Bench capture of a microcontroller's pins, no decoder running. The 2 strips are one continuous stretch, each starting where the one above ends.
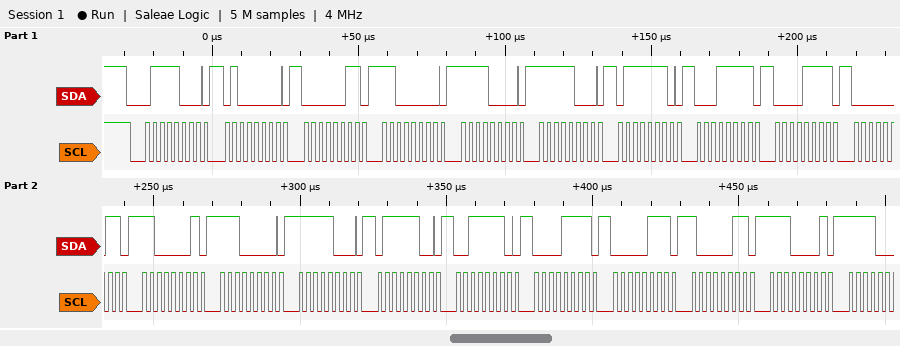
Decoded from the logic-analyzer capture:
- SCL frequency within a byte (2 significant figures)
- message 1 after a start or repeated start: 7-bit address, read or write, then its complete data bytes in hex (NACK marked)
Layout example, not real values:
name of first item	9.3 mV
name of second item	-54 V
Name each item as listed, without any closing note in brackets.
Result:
SCL frequency within a byte	400 kHz
message 1 after a start or repeated start: 7-bit address, read or write, then its complete data bytes in hex	0x3C write: 40 03 C0 F0 F8 7E 1F 0F 03 C1 E0 F8 7C 3E 0F 07 83 E1
